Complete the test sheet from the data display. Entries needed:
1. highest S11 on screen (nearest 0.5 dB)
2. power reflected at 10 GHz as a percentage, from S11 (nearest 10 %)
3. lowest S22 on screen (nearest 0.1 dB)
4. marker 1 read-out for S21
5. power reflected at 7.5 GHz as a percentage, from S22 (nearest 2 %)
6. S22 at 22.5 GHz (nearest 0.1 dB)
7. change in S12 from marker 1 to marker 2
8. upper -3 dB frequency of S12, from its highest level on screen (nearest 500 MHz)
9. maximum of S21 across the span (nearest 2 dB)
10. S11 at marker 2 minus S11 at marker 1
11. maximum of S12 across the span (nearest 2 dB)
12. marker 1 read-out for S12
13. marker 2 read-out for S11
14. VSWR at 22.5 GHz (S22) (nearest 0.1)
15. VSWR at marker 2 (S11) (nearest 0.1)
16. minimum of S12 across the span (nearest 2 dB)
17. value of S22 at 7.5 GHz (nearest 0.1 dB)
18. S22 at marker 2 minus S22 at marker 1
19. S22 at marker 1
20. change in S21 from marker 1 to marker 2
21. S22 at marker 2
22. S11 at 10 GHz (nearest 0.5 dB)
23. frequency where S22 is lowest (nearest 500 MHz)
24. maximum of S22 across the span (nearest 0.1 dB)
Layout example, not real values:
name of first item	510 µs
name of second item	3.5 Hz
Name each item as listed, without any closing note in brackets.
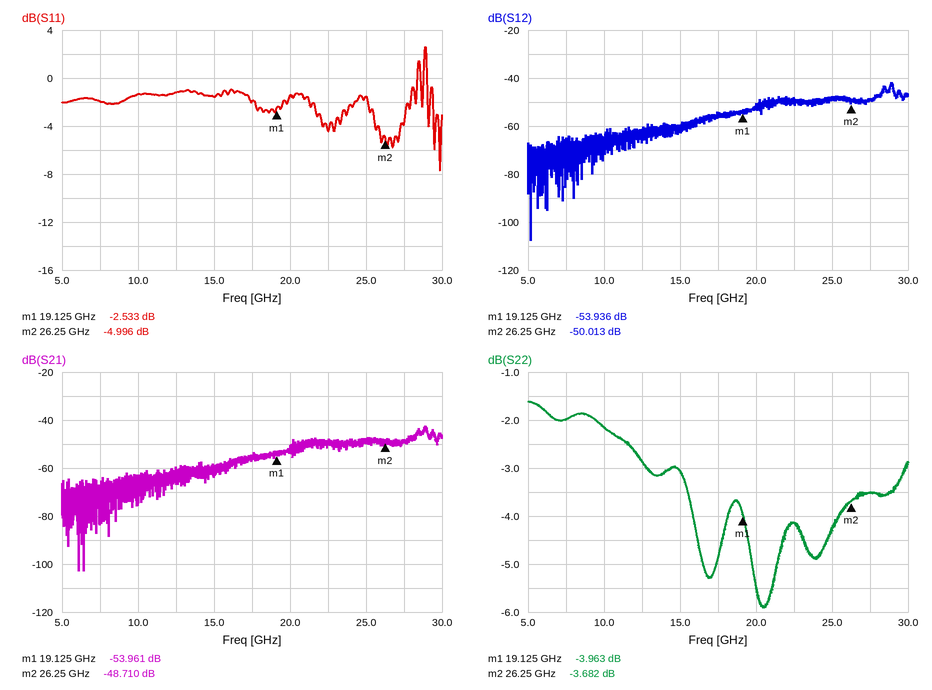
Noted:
highest S11 on screen	2.5 dB
power reflected at 10 GHz as a percentage, from S11	70 %
lowest S22 on screen	-5.9 dB
marker 1 read-out for S21	-53.961 dB
power reflected at 7.5 GHz as a percentage, from S22	64 %
S22 at 22.5 GHz	-4.1 dB
change in S12 from marker 1 to marker 2	3.923 dB
upper -3 dB frequency of S12, from its highest level on screen	29.0 GHz
maximum of S21 across the span	-42 dB
S11 at marker 2 minus S11 at marker 1	-2.463 dB
maximum of S12 across the span	-42 dB
marker 1 read-out for S12	-53.936 dB
marker 2 read-out for S11	-4.996 dB
VSWR at 22.5 GHz (S22)	4.3
VSWR at marker 2 (S11)	3.6
minimum of S12 across the span	-108 dB
value of S22 at 7.5 GHz	-2.0 dB
S22 at marker 2 minus S22 at marker 1	0.281 dB
S22 at marker 1	-3.963 dB
change in S21 from marker 1 to marker 2	5.251 dB
S22 at marker 2	-3.682 dB
S11 at 10 GHz	-1.5 dB
frequency where S22 is lowest	20.5 GHz
maximum of S22 across the span	-1.6 dB
